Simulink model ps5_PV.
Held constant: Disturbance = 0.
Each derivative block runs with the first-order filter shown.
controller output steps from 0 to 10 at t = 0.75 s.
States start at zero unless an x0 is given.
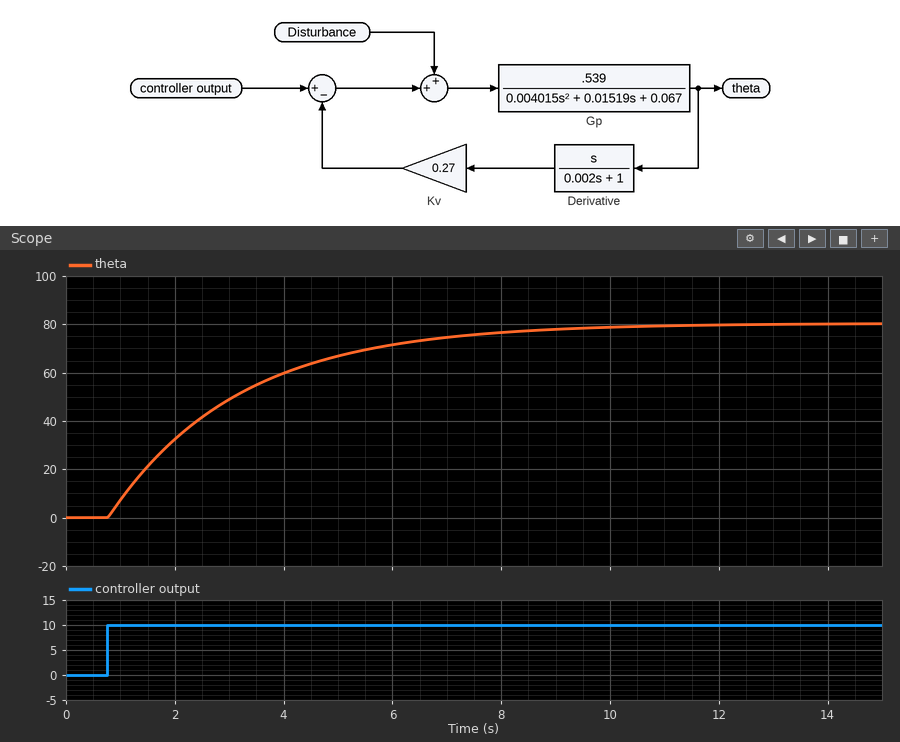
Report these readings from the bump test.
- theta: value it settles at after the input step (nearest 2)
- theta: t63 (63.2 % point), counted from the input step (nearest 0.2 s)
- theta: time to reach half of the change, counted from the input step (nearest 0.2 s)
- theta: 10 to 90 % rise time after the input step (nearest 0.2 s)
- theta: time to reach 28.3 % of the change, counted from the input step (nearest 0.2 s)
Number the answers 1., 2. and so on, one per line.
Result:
1. 80
2. 2.4 s
3. 1.6 s
4. 5.2 s
5. 0.8 s
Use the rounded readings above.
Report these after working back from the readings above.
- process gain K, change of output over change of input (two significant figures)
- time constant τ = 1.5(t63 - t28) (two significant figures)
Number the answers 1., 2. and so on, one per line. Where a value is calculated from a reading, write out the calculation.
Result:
1. (80 - 0) / 10 = 8.0
2. 1.5 × (2.4 - 0.8) = 2.4 s
